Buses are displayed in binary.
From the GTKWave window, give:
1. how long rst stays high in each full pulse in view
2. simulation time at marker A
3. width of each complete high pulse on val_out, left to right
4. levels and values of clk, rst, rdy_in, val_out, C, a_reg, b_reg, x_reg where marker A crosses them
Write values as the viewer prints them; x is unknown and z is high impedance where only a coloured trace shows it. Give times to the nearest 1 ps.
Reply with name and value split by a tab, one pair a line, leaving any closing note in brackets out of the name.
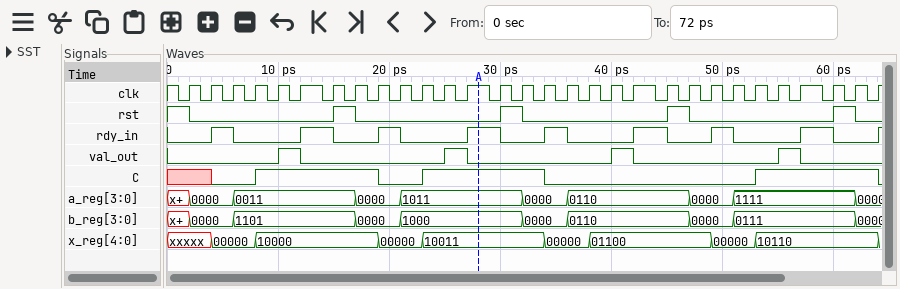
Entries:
how long rst stays high in each full pulse in view	2 ps, 2 ps, 2 ps, 2 ps
simulation time at marker A	28 ps
width of each complete high pulse on val_out, left to right	2 ps, 2 ps, 2 ps, 2 ps
levels and values of clk, rst, rdy_in, val_out, C, a_reg, b_reg, x_reg where marker A crosses them	clk=1, rst=0, rdy_in=1, val_out=0, C=1, a_reg=1011, b_reg=1000, x_reg=10011
